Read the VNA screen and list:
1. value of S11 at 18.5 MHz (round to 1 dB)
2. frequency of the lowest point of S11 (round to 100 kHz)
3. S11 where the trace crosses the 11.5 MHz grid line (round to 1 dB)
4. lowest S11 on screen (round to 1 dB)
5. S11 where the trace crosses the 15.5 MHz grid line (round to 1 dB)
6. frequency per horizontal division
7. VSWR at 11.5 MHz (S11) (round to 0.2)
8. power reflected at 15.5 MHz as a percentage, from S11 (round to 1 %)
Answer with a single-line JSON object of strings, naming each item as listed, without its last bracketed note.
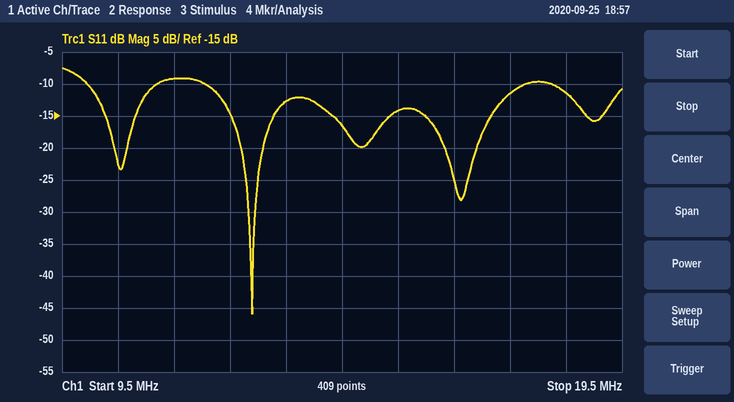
{"value of S11 at 18.5 MHz": "-11 dB", "frequency of the lowest point of S11": "12.9 MHz", "S11 where the trace crosses the 11.5 MHz grid line": "-9 dB", "lowest S11 on screen": "-46 dB", "S11 where the trace crosses the 15.5 MHz grid line": "-14 dB", "frequency per horizontal division": "1 MHz", "VSWR at 11.5 MHz (S11)": "2.0", "power reflected at 15.5 MHz as a percentage, from S11": "4 %"}
